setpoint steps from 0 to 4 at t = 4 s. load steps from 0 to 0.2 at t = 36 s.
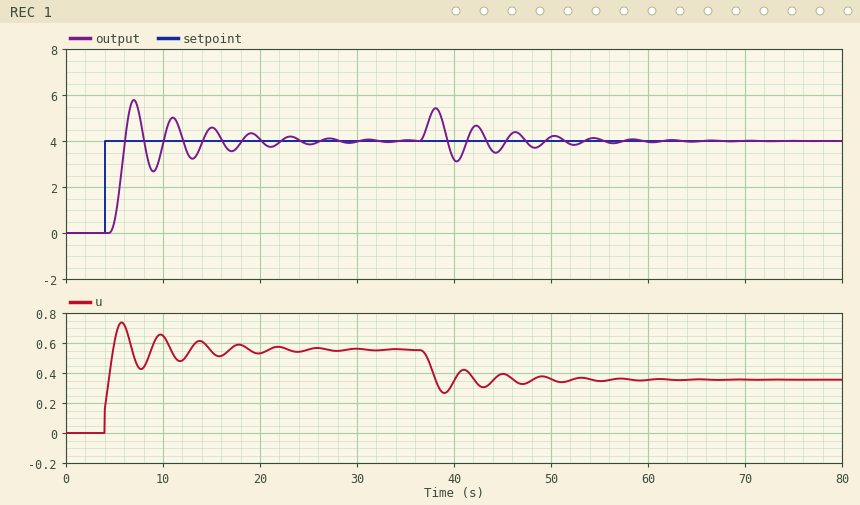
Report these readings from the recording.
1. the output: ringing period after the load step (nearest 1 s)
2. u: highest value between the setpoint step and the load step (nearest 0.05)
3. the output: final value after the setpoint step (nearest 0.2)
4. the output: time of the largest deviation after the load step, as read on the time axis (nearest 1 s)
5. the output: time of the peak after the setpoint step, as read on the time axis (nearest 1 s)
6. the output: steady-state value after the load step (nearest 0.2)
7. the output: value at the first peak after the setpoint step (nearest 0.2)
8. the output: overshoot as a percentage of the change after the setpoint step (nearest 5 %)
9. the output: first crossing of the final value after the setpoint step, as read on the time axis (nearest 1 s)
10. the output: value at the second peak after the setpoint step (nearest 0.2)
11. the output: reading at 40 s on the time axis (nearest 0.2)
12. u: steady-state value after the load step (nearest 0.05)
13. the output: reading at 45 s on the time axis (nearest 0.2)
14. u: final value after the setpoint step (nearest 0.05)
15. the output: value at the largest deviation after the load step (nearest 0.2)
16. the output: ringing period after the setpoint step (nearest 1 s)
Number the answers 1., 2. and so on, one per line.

1. 4 s
2. 0.75
3. 4.0
4. 38 s
5. 7 s
6. 4.0
7. 5.8
8. 45 %
9. 6 s
10. 5.0
11. 3.2
12. 0.35
13. 3.8
14. 0.55
15. 5.4
16. 4 s
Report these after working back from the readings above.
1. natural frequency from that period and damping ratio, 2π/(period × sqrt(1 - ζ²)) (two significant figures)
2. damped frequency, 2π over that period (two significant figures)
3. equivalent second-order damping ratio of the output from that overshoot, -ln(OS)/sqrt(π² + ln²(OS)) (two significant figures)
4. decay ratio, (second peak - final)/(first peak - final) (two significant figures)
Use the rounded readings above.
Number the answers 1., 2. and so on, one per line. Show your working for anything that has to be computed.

1. 2π / (4 × sqrt(1 - 0.25²)) = 1.6 rad/s
2. 2π / 4 = 1.6 rad/s
3. ln(0.45) = -0.799; 0.799 / sqrt(9.870 + 0.638) = 0.25
4. (5 - 4) / (5.8 - 4) = 0.56
